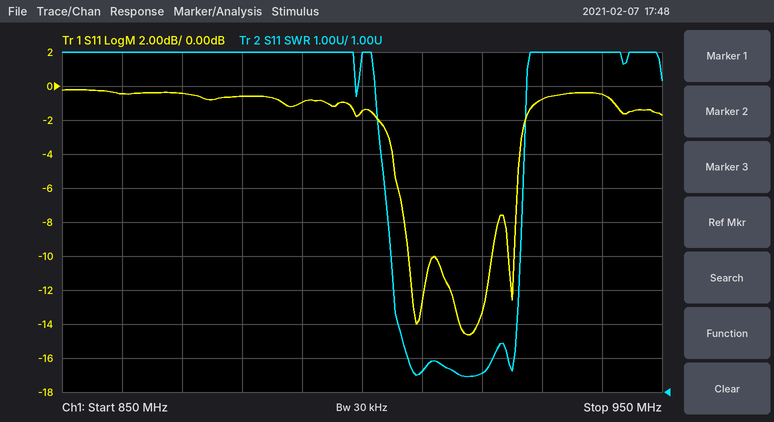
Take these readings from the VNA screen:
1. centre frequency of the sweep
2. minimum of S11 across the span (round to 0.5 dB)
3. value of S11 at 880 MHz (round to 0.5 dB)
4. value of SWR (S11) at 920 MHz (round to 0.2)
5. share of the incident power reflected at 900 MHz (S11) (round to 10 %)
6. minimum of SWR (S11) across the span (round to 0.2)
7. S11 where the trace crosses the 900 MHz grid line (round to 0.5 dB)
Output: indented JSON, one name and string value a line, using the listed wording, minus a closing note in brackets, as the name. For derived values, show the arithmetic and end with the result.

{
  "centre frequency of the sweep": "900 MHz",
  "minimum of S11 across the span": "-14.5 dB",
  "value of S11 at 880 MHz": "-0.5 dB",
  "value of SWR (S11) at 920 MHz": "1.6",
  "share of the incident power reflected at 900 MHz (S11)": "10^(-1.5/10) ≈ 70.8 %, so 70 % to the nearest 10 %",
  "minimum of SWR (S11) across the span": "1.4",
  "S11 where the trace crosses the 900 MHz grid line": "-1.5 dB"
}
